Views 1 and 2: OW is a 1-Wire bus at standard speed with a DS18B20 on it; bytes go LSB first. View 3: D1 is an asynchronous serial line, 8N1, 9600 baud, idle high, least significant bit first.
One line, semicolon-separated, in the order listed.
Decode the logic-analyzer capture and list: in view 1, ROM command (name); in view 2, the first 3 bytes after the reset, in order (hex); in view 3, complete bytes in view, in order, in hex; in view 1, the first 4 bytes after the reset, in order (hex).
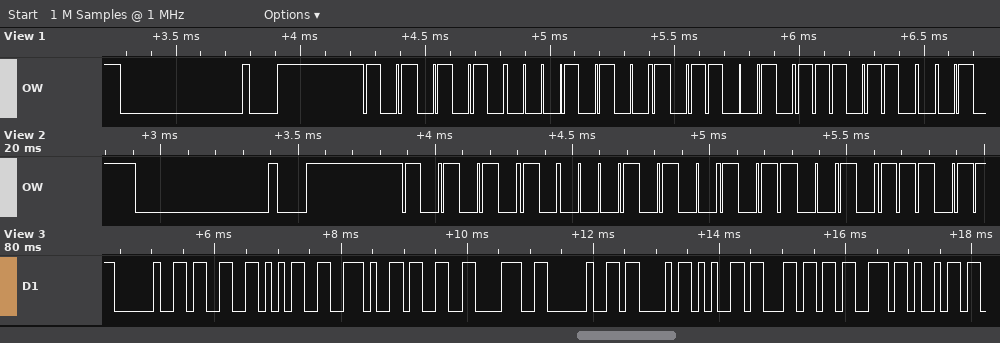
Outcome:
Match ROM; 55 28 4D; 20 33 35 2E 33 38 20 43 65 6C 73 69; 55 28 4D 37
